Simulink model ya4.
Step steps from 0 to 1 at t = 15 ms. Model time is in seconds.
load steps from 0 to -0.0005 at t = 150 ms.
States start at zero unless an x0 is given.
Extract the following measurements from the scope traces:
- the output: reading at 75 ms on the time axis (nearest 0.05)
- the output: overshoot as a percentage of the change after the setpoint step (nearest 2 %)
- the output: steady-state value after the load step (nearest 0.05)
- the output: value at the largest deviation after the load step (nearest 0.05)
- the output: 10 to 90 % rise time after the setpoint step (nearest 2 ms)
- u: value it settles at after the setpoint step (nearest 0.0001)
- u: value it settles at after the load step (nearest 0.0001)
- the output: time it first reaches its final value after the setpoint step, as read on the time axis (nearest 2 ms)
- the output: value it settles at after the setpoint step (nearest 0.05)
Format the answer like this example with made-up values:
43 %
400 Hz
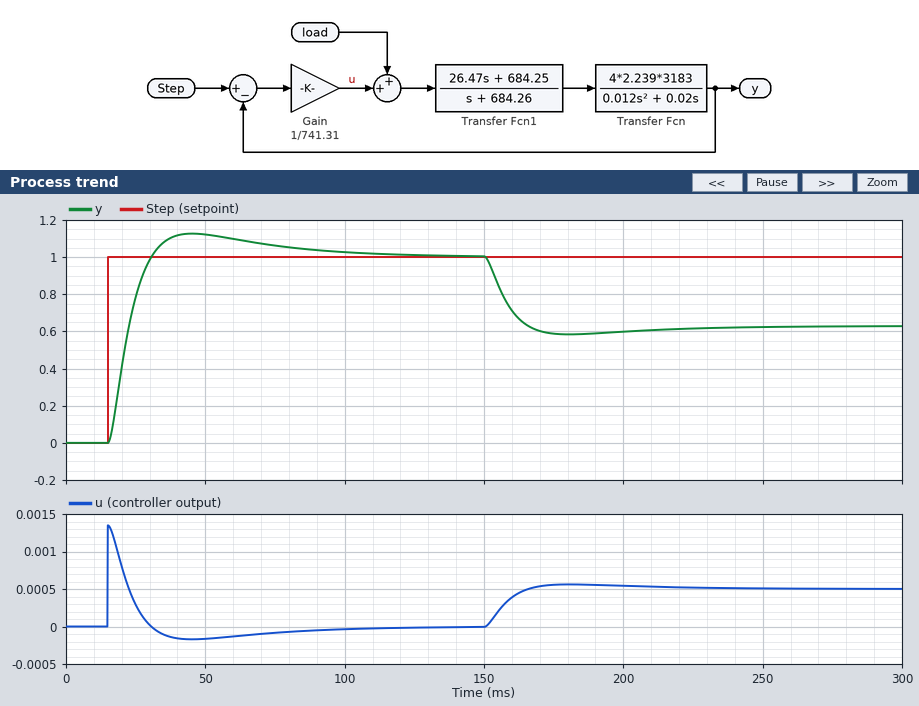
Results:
1.05
12 %
0.65
0.60
10 ms
0.0000
0.0005
30 ms
1.00
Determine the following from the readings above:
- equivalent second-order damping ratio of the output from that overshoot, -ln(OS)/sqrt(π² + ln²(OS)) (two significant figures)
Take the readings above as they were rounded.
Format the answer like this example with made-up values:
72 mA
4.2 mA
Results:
0.56
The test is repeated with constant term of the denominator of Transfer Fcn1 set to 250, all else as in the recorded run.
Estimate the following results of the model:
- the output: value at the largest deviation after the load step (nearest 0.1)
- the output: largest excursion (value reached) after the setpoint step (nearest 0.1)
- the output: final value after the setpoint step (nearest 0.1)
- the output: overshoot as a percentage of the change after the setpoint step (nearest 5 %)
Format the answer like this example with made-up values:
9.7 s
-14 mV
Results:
0.5
1.3
1.0
35 %
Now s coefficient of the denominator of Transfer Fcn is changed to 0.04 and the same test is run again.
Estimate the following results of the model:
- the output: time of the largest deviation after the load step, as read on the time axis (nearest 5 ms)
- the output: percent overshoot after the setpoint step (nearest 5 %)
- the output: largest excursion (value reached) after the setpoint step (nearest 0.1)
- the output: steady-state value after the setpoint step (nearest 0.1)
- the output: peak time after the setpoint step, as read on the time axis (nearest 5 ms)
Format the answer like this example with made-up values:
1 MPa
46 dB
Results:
180 ms
10 %
1.1
1.0
45 ms
